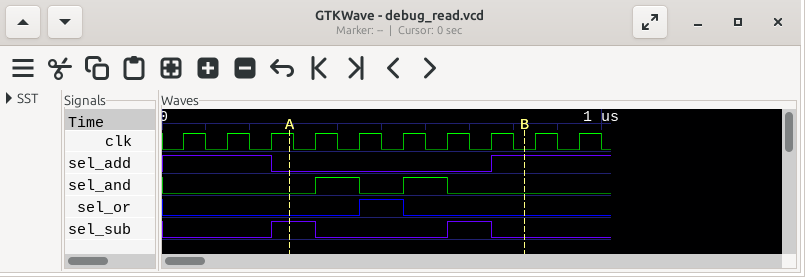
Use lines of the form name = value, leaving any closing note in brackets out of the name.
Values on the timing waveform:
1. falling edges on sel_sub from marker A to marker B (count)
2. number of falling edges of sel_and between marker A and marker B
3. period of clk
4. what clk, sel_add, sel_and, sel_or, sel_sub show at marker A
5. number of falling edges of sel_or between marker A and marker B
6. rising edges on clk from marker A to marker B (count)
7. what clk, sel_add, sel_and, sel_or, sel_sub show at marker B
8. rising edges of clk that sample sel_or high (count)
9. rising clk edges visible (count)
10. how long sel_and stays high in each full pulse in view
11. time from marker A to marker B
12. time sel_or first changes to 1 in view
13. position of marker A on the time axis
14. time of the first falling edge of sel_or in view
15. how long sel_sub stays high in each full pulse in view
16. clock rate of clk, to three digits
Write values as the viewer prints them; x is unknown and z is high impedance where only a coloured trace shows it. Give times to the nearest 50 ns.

falling edges on sel_sub from marker A to marker B = 2
number of falling edges of sel_and between marker A and marker B = 2
period of clk = 100 ns
what clk, sel_add, sel_and, sel_or, sel_sub show at marker A = clk=1, sel_add=0, sel_and=0, sel_or=0, sel_sub=1
number of falling edges of sel_or between marker A and marker B = 1
rising edges on clk from marker A to marker B = 5
what clk, sel_add, sel_and, sel_or, sel_sub show at marker B = clk=0, sel_add=1, sel_and=0, sel_or=0, sel_sub=0
rising edges of clk that sample sel_or high = 1
rising clk edges visible = 10
how long sel_and stays high in each full pulse in view = 100 ns, 100 ns
time from marker A to marker B = 550 ns
time sel_or first changes to 1 in view = 450 ns
position of marker A on the time axis = 300 ns
time of the first falling edge of sel_or in view = 550 ns
how long sel_sub stays high in each full pulse in view = 100 ns, 100 ns
clock rate of clk, to three digits = 10.0 MHz
